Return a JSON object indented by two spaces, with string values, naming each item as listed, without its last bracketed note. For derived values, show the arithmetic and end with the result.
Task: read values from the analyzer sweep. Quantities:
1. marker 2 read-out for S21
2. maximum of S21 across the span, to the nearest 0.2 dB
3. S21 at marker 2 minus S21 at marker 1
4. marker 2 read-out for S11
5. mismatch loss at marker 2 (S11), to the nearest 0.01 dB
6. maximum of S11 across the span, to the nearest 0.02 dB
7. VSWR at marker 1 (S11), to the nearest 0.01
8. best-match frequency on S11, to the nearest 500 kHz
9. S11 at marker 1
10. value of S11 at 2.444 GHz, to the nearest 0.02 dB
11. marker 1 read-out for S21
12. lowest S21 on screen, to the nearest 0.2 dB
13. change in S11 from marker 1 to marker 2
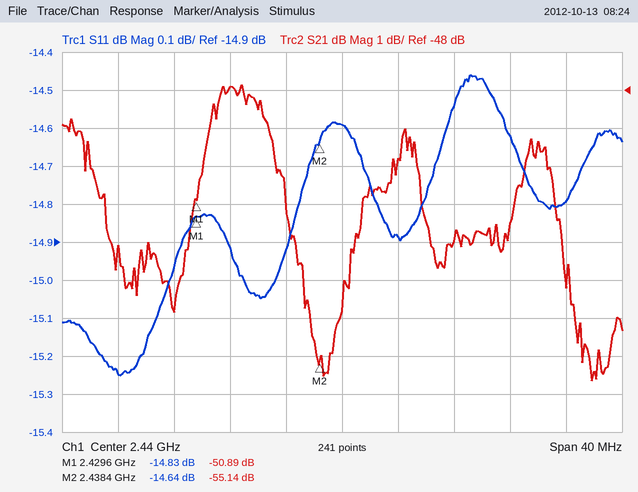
{
  "marker 2 read-out for S21": "-55.14 dB",
  "maximum of S21 across the span, to the nearest 0.2 dB": "-47.8 dB",
  "S21 at marker 2 minus S21 at marker 1": "-55.14 − (-50.89) = -4.25 dB",
  "marker 2 read-out for S11": "-14.64 dB",
  "mismatch loss at marker 2 (S11), to the nearest 0.01 dB": "−10 log10(1 − 10^(-14.64/10)) ≈ 0.15 dB",
  "maximum of S11 across the span, to the nearest 0.02 dB": "-14.46 dB",
  "VSWR at marker 1 (S11), to the nearest 0.01": "(1 + 0.1813)/(1 − 0.1813) ≈ 1.44",
  "best-match frequency on S11, to the nearest 500 kHz": "2.4240 GHz",
  "S11 at marker 1": "-14.83 dB",
  "value of S11 at 2.444 GHz, to the nearest 0.02 dB": "-14.88 dB",
  "marker 1 read-out for S21": "-50.89 dB",
  "lowest S21 on screen, to the nearest 0.2 dB": "-55.6 dB",
  "change in S11 from marker 1 to marker 2": "-14.64 − (-14.83) = 0.19 dB"
}
